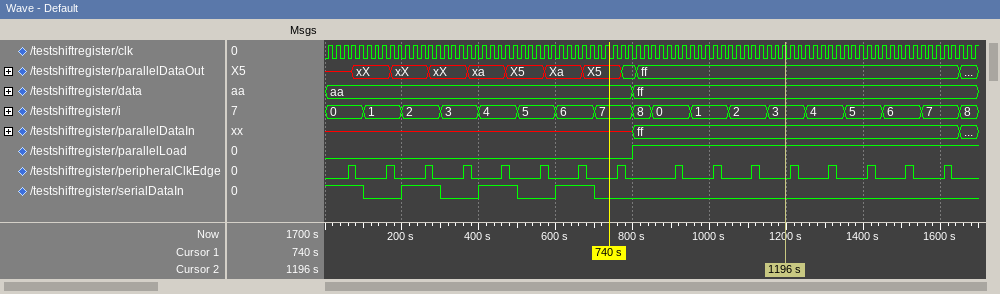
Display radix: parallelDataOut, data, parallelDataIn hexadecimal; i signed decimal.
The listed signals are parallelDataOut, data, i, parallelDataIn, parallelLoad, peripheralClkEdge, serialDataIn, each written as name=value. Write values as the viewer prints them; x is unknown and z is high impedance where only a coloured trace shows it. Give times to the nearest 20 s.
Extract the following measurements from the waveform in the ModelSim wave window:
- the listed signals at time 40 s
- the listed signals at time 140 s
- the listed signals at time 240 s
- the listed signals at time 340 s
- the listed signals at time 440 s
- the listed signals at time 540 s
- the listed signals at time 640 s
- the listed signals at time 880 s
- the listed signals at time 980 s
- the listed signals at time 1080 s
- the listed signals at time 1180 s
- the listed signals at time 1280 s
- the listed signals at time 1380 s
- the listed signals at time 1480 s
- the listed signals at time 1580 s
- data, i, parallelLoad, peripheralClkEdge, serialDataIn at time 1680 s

parallelDataOut=x, data=aa, i=0, parallelDataIn=x, parallelLoad=0, peripheralClkEdge=0, serialDataIn=1
parallelDataOut=xX, data=aa, i=1, parallelDataIn=x, parallelLoad=0, peripheralClkEdge=0, serialDataIn=0
parallelDataOut=xX, data=aa, i=2, parallelDataIn=x, parallelLoad=0, peripheralClkEdge=0, serialDataIn=1
parallelDataOut=xX, data=aa, i=3, parallelDataIn=x, parallelLoad=0, peripheralClkEdge=0, serialDataIn=0
parallelDataOut=xa, data=aa, i=4, parallelDataIn=x, parallelLoad=0, peripheralClkEdge=0, serialDataIn=1
parallelDataOut=X5, data=aa, i=5, parallelDataIn=x, parallelLoad=0, peripheralClkEdge=0, serialDataIn=0
parallelDataOut=Xa, data=aa, i=6, parallelDataIn=x, parallelLoad=0, peripheralClkEdge=0, serialDataIn=1
parallelDataOut=ff, data=ff, i=0, parallelDataIn=ff, parallelLoad=1, peripheralClkEdge=0, serialDataIn=0
parallelDataOut=ff, data=ff, i=1, parallelDataIn=ff, parallelLoad=1, peripheralClkEdge=0, serialDataIn=0
parallelDataOut=ff, data=ff, i=2, parallelDataIn=ff, parallelLoad=1, peripheralClkEdge=0, serialDataIn=0
parallelDataOut=ff, data=ff, i=3, parallelDataIn=ff, parallelLoad=1, peripheralClkEdge=0, serialDataIn=0
parallelDataOut=ff, data=ff, i=4, parallelDataIn=ff, parallelLoad=1, peripheralClkEdge=0, serialDataIn=0
parallelDataOut=ff, data=ff, i=5, parallelDataIn=ff, parallelLoad=1, peripheralClkEdge=0, serialDataIn=0
parallelDataOut=ff, data=ff, i=6, parallelDataIn=ff, parallelLoad=1, peripheralClkEdge=0, serialDataIn=0
parallelDataOut=ff, data=ff, i=7, parallelDataIn=ff, parallelLoad=1, peripheralClkEdge=0, serialDataIn=0
data=ff, i=8, parallelLoad=1, peripheralClkEdge=0, serialDataIn=0
